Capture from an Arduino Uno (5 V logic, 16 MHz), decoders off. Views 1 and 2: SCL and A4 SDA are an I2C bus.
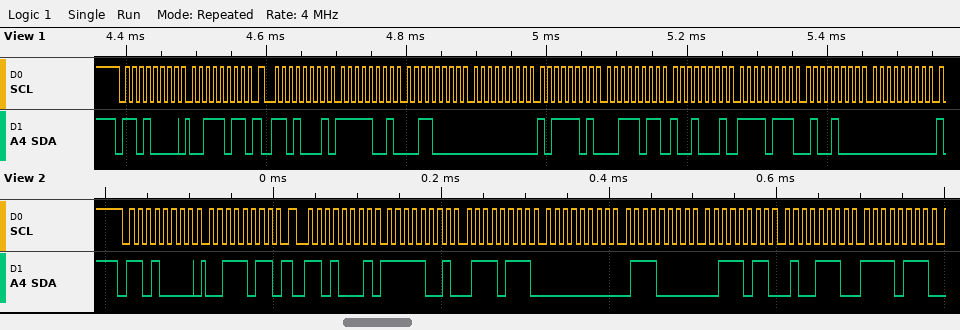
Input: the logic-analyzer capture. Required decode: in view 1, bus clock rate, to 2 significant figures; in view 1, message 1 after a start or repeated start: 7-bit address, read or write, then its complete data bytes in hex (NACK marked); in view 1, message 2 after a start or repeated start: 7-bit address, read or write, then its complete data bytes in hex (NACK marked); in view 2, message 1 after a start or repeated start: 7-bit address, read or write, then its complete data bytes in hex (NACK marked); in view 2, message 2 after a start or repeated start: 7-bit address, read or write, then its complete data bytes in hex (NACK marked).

100 kHz
0x68 write: 3B
0x68 read: F9 30 00 BD 3B 91 F7 48 00
0x68 write: 3B
0x68 read: F9 77 00 70 3B 4E F7
